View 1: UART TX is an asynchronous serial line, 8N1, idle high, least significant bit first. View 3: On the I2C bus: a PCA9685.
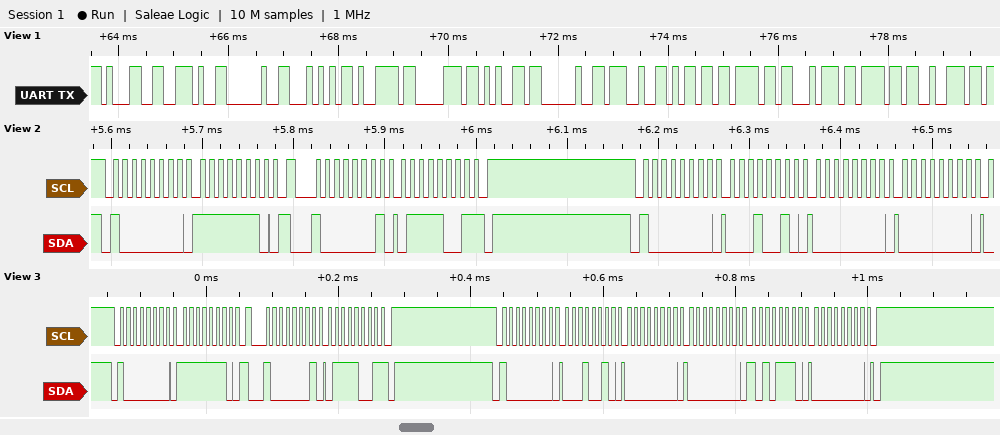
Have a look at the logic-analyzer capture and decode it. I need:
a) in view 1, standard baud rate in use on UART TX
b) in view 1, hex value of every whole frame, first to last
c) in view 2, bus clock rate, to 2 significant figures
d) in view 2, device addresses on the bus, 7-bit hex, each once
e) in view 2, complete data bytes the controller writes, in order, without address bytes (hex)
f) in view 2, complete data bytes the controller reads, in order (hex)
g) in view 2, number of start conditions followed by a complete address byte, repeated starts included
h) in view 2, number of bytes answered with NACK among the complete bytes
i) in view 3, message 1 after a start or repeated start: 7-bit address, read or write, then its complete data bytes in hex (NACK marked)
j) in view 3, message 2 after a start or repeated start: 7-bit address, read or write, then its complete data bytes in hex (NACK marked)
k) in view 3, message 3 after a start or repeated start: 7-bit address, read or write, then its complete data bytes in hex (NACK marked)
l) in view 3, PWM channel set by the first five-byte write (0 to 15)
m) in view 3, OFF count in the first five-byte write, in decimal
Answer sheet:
9600 baud
0x31 0x2E 0x20 0x54 0x79 0x70 0x65 0x20 0x27 0x6D 0x6F 0x74 0x6F 0x72
100 kHz
0x40
FE 12 00 00
79
3
1
0x40 write: FE
0x40 read: 79 NACK
0x40 write: 12 00 00 AE 00
3
174
